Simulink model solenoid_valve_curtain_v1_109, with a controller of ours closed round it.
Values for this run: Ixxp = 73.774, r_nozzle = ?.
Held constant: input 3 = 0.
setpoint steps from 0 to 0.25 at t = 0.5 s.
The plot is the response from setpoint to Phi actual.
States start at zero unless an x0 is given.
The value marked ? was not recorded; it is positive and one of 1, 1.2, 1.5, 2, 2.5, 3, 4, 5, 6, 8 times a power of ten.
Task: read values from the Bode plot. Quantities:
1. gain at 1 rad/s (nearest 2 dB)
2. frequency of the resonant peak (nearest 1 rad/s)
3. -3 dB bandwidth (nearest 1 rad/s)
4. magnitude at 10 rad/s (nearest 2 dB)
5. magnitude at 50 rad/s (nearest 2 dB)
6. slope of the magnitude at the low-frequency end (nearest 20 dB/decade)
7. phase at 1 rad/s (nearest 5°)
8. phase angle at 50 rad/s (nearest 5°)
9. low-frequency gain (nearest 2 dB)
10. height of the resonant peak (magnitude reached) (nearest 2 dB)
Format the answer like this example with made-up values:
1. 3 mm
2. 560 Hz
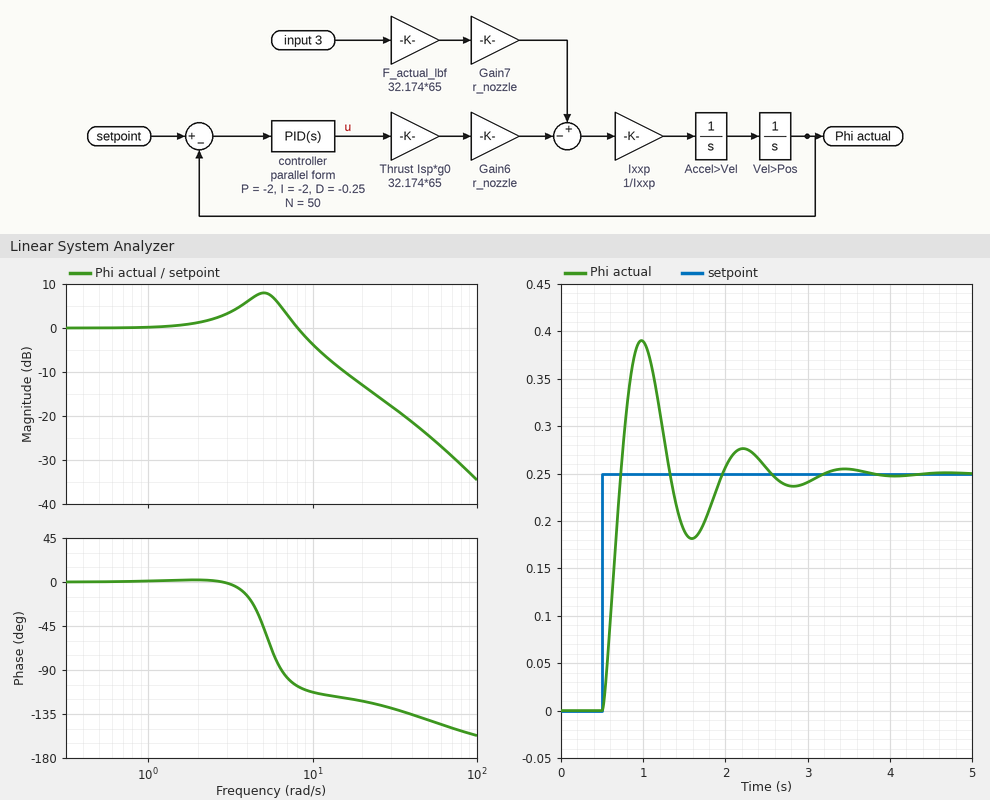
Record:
1. 0 dB
2. 5 rad/s
3. 10 rad/s
4. -4 dB
5. -24 dB
6. 0 dB/decade
7. 0°
8. -140°
9. 0 dB
10. 8 dB
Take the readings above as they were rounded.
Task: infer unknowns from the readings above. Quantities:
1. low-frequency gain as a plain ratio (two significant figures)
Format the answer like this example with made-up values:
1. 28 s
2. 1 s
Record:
1. 1.0
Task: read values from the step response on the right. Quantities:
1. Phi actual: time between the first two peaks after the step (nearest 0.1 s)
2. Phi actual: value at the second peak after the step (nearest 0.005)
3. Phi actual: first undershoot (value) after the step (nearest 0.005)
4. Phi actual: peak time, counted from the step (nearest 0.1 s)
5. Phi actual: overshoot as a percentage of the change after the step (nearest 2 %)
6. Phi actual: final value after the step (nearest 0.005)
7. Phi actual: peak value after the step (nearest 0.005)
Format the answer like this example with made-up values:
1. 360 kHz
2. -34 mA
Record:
1. 1.2 s
2. 0.275
3. 0.180
4. 0.5 s
5. 56 %
6. 0.250
7. 0.390
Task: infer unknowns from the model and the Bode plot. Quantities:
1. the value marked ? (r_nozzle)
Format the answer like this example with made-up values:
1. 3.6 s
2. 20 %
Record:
1. 0.5
